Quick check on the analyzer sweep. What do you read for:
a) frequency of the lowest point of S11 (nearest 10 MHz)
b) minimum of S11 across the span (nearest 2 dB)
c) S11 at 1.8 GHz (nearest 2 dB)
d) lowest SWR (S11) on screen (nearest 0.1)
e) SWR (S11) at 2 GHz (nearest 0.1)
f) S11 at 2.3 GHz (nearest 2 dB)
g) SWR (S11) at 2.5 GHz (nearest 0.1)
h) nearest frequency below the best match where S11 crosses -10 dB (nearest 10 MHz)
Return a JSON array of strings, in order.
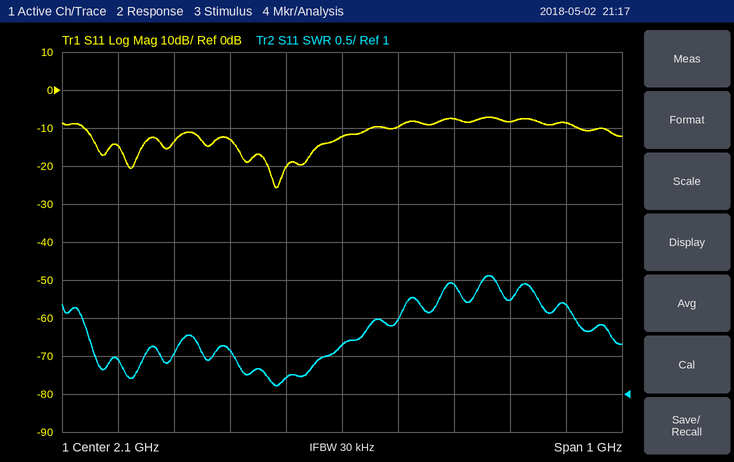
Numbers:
["1.98 GHz", "-26 dB", "-14 dB", "1.1", "1.2", "-8 dB", "2.2", "1.64 GHz"]
